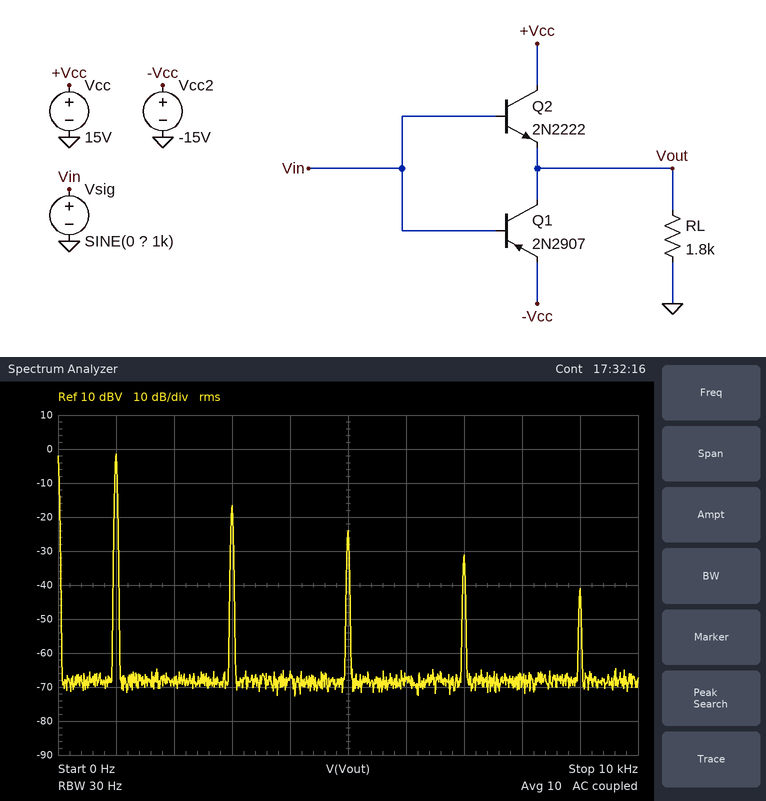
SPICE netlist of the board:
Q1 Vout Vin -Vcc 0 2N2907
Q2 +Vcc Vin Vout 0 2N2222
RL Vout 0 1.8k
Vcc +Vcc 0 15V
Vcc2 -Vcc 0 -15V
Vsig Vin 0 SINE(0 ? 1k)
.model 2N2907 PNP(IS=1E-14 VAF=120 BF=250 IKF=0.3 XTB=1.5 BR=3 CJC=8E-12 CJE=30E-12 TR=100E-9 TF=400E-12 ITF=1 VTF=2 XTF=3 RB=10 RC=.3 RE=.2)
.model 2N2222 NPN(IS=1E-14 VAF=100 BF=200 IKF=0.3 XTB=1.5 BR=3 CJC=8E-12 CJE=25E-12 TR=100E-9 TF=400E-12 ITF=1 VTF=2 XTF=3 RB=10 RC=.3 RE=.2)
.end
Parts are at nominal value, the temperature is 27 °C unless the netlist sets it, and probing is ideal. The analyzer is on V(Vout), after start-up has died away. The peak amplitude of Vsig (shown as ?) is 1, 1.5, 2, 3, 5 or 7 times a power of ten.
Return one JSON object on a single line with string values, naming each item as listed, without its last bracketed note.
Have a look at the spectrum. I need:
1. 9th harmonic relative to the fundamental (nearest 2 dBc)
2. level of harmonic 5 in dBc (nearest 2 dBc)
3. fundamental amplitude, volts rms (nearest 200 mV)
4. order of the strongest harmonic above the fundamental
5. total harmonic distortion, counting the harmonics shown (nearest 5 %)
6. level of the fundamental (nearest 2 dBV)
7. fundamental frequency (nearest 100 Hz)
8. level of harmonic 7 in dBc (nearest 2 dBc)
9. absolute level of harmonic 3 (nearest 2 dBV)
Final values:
{"9th harmonic relative to the fundamental": "-40 dBc", "level of harmonic 5 in dBc": "-22 dBc", "fundamental amplitude, volts rms": "800 mV", "order of the strongest harmonic above the fundamental": "3", "total harmonic distortion, counting the harmonics shown": "20 %", "level of the fundamental": "-2 dBV", "fundamental frequency": "1.0 kHz", "level of harmonic 7 in dBc": "-30 dBc", "absolute level of harmonic 3": "-16 dBV"}
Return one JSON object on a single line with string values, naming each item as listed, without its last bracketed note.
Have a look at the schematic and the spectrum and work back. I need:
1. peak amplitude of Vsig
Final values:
{"peak amplitude of Vsig": "2 V"}
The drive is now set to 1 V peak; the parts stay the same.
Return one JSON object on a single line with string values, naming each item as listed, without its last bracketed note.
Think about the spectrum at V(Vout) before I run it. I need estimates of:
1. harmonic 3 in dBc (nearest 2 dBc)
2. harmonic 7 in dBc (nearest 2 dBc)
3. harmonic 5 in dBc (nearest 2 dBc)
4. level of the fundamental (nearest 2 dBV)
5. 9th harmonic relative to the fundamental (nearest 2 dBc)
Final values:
{"harmonic 3 in dBc": "-8 dBc", "harmonic 7 in dBc": "-28 dBc", "harmonic 5 in dBc": "-30 dBc", "level of the fundamental": "-14 dBV", "9th harmonic relative to the fundamental": "-32 dBc"}
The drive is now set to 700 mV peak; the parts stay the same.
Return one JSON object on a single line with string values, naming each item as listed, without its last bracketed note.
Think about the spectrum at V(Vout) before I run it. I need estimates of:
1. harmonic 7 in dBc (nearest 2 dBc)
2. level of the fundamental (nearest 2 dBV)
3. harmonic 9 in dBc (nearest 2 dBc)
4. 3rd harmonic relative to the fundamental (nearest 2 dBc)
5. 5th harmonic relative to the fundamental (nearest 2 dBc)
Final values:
{"harmonic 7 in dBc": "-32 dBc", "level of the fundamental": "-26 dBV", "harmonic 9 in dBc": "-28 dBc", "3rd harmonic relative to the fundamental": "-4 dBc", "5th harmonic relative to the fundamental": "-14 dBc"}
